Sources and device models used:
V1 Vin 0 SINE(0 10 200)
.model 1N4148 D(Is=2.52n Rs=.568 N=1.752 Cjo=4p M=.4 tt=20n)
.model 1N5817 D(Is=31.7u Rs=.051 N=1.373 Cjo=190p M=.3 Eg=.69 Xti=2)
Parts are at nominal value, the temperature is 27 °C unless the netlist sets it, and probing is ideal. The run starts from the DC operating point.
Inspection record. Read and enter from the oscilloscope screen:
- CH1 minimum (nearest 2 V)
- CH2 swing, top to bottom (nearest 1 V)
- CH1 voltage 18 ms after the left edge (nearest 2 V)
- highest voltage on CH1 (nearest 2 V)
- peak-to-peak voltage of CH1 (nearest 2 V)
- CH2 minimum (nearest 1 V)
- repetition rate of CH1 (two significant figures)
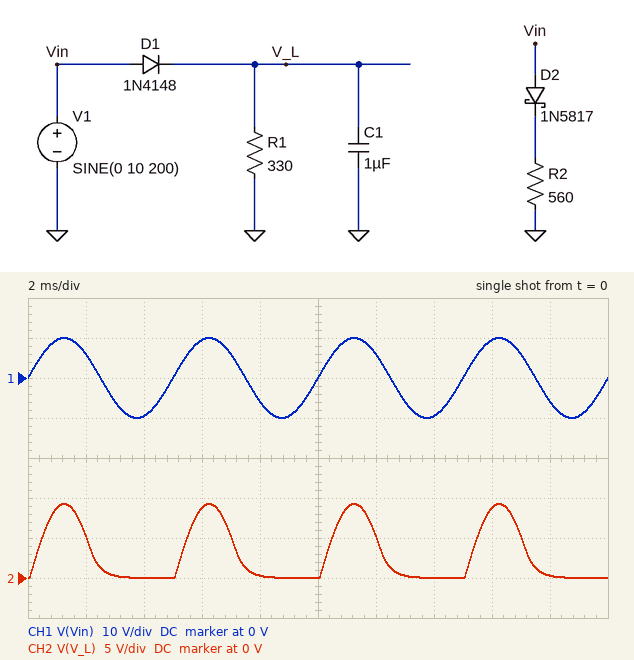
-10 V
9 V
-6 V
10 V
20 V
0 V
200 Hz
